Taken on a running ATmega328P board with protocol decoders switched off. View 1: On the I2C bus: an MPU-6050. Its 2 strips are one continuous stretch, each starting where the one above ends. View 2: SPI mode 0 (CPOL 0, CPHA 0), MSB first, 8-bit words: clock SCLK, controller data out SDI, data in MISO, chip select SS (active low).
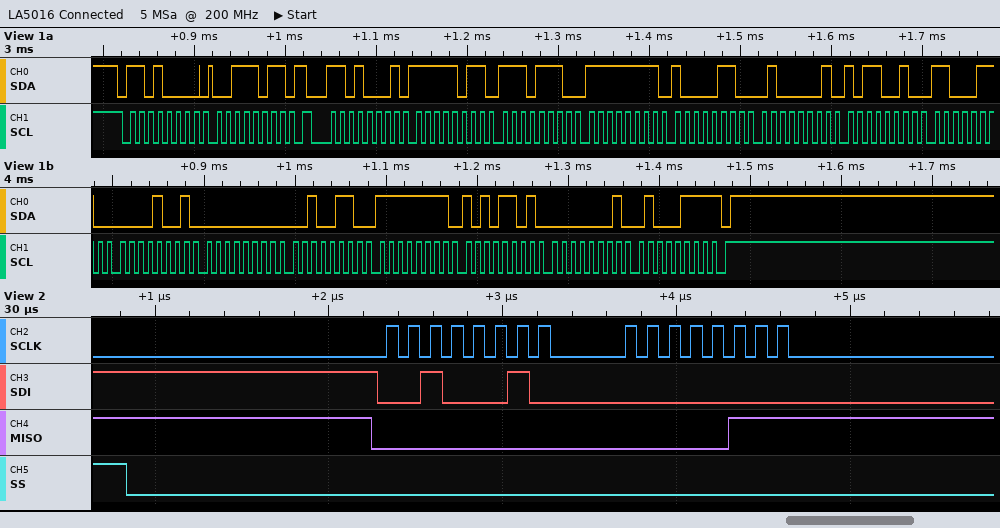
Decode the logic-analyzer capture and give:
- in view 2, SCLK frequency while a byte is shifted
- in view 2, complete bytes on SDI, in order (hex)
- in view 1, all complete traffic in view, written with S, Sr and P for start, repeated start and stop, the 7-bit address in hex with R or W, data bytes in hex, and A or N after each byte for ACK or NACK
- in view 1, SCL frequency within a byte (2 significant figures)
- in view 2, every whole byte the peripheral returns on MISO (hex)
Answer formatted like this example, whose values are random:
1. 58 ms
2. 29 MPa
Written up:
1. 8 MHz
2. 0x22 0x00
3. S 68W A 3B A Sr 68R A FB A EE A FF A 86 A 41 A B2 A C6 A 09 A 00 A 26 A FF A AD A 01 A 47 N P
4. 100 kHz
5. 0x00 0x07
